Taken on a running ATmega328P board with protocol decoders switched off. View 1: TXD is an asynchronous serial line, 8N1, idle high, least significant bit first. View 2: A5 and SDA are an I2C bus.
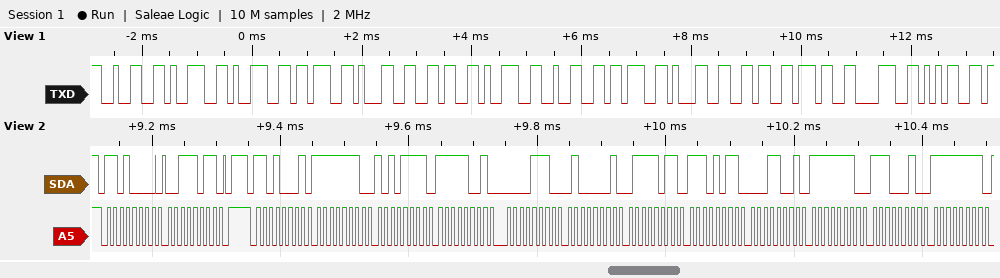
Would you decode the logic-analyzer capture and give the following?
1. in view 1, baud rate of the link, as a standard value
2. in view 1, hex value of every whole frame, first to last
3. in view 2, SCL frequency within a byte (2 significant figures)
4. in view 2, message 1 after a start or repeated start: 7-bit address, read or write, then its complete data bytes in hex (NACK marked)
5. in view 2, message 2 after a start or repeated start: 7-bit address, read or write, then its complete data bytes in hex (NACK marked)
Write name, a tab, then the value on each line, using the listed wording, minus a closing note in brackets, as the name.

in view 1, baud rate of the link, as a standard value	9600 baud
in view 1, hex value of every whole frame, first to last	32 39 39 3B 31 36 39 32 3B 31 36 37 38 35
in view 2, SCL frequency within a byte	100 kHz
in view 2, message 1 after a start or repeated start: 7-bit address, read or write, then its complete data bytes in hex	0x68 write: 3B
in view 2, message 2 after a start or repeated start: 7-bit address, read or write, then its complete data bytes in hex	0x68 read: FE AF F9 0E 41 7B EB 19 FE E2 FF
